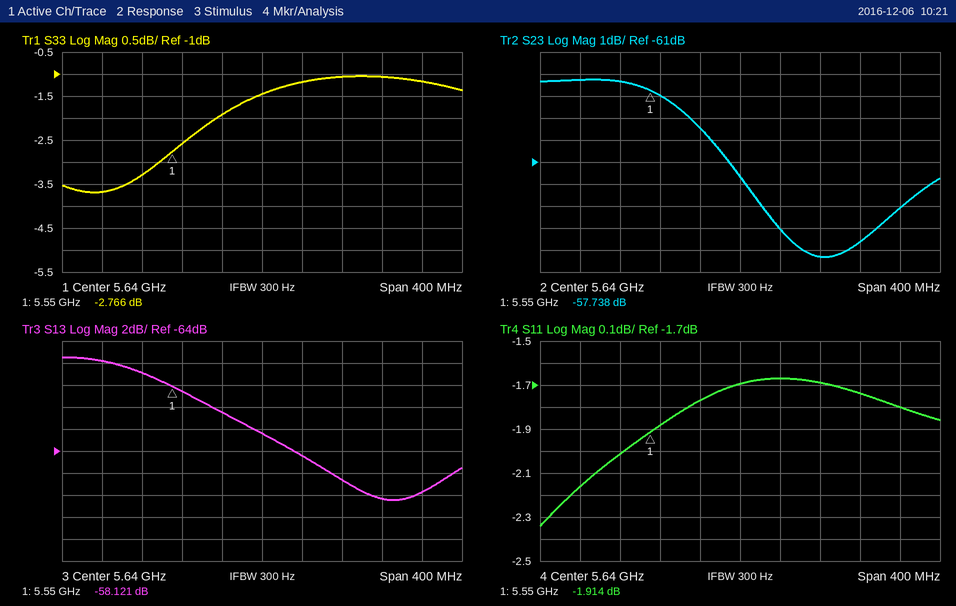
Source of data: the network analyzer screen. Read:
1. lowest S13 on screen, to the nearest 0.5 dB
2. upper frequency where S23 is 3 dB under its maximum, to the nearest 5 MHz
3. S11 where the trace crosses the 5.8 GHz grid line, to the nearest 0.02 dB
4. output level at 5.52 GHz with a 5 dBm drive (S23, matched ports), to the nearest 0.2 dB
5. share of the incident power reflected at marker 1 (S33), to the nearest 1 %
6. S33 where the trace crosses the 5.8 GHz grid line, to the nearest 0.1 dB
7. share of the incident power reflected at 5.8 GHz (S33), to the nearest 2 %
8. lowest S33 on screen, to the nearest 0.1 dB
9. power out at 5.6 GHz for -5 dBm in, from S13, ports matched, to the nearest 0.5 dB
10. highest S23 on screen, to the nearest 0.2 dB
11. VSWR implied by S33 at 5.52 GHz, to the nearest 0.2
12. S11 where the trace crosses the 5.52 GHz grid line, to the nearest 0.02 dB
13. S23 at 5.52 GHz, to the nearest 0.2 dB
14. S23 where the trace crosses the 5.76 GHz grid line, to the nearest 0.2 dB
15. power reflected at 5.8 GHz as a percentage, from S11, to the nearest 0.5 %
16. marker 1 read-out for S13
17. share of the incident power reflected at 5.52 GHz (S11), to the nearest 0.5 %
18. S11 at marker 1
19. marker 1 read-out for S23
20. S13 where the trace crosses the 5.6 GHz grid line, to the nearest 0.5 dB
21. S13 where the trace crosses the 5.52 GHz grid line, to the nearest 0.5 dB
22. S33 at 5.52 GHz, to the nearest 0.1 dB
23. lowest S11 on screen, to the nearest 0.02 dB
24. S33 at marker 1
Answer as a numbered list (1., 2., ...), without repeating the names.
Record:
1. -68.5 dB
2. 5.615 GHz
3. -1.80 dB
4. -52.4 dBm
5. 53 %
6. -1.2 dB
7. 76 %
8. -3.7 dB
9. -65.5 dBm
10. -57.2 dB
11. 5.4
12. -2.02 dB
13. -57.4 dB
14. -64.6 dB
15. 66.0 %
16. -58.121 dB
17. 63.0 %
18. -1.914 dB
19. -57.738 dB
20. -60.5 dB
21. -57.0 dB
22. -3.3 dB
23. -2.34 dB
24. -2.766 dB
